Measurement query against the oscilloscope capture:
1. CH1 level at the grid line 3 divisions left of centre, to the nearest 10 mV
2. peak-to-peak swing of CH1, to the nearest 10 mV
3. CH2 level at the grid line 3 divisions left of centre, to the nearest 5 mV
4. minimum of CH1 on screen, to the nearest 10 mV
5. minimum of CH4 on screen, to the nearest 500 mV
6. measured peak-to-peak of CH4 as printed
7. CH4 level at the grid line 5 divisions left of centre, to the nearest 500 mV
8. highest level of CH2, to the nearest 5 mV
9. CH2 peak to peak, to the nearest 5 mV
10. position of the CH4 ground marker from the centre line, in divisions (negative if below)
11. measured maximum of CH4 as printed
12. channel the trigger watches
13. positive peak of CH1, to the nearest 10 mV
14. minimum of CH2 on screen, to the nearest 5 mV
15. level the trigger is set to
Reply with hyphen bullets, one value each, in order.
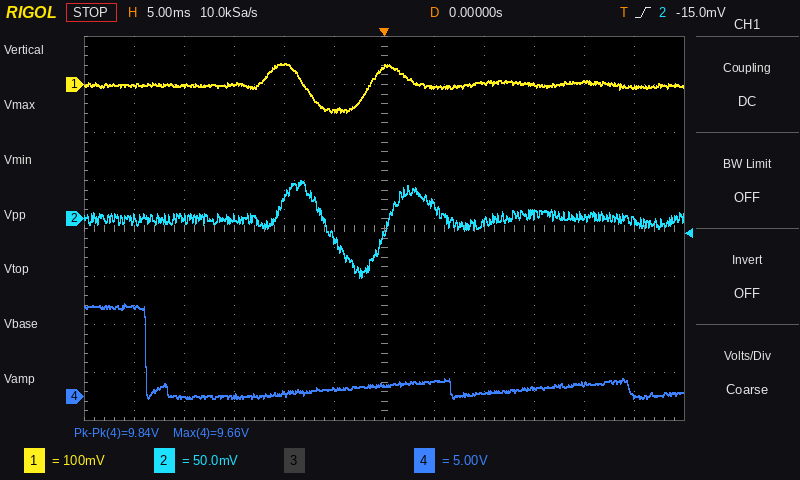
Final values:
- 0 mV
- 100 mV
- 0 mV
- -60 mV
- 0.0 V
- 9.84 V
- 9.5 V
- 40 mV
- 100 mV
- -3.5 div
- 9.66 V
- CH2
- 40 mV
- -60 mV
- -15.0 mV
